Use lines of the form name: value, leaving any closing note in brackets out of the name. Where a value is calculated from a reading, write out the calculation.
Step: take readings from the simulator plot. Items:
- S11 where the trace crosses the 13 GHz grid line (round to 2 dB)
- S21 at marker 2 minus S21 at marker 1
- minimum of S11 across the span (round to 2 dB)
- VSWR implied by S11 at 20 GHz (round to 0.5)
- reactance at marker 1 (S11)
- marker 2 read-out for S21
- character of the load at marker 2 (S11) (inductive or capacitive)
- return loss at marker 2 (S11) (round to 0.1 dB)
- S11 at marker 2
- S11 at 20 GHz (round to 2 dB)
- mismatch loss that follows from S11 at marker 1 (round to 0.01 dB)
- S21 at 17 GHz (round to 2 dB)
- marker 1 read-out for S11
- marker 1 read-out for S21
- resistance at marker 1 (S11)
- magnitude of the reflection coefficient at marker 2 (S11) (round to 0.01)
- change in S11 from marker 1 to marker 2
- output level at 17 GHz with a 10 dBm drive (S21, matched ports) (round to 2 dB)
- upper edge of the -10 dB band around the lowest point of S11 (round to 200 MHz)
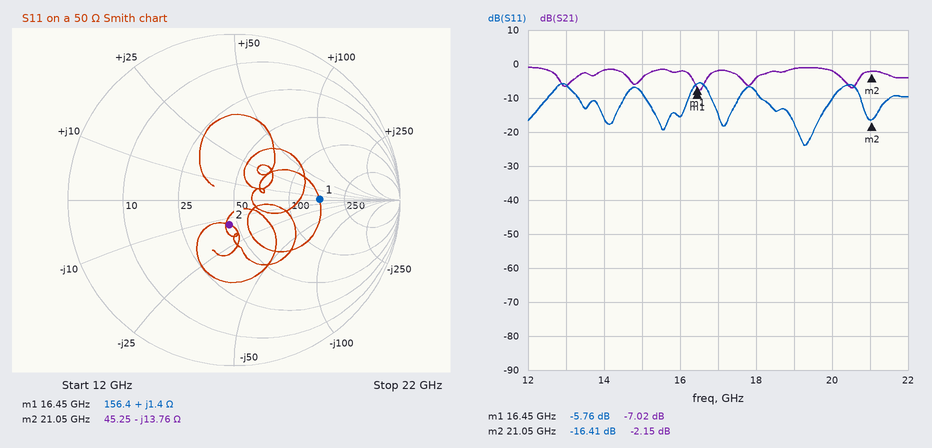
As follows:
S11 where the trace crosses the 13 GHz grid line: -6 dB
S21 at marker 2 minus S21 at marker 1: -2.15 − (-7.02) = 4.87 dB
minimum of S11 across the span: -24 dB
VSWR implied by S11 at 20 GHz: |Γ| = 10^(-10/20) = 0.3162; VSWR = (1 + 0.3162)/(1 − 0.3162) ≈ 1.92, so 2.0 to the nearest 0.5
reactance at marker 1: +1.4 Ω
marker 2 read-out for S21: -2.15 dB
character of the load at marker 2 (S11): capacitive
return loss at marker 2 (S11): 16.4 dB
S11 at marker 2: -16.41 dB
S11 at 20 GHz: -10 dB
mismatch loss that follows from S11 at marker 1: −10 log10(1 − 10^(-5.76/10)) ≈ 1.34 dB
S21 at 17 GHz: -2 dB
marker 1 read-out for S11: -5.76 dB
marker 1 read-out for S21: -7.02 dB
resistance at marker 1: 156.4 Ω
magnitude of the reflection coefficient at marker 2 (S11): 10^(-16.41/20) ≈ 0.15
change in S11 from marker 1 to marker 2: -16.41 − (-5.76) = -10.65 dB
output level at 17 GHz with a 10 dBm drive (S21, matched ports): 10 dBm + (-2 dB) = 8 dBm
upper edge of the -10 dB band around the lowest point of S11: 20.0 GHz
